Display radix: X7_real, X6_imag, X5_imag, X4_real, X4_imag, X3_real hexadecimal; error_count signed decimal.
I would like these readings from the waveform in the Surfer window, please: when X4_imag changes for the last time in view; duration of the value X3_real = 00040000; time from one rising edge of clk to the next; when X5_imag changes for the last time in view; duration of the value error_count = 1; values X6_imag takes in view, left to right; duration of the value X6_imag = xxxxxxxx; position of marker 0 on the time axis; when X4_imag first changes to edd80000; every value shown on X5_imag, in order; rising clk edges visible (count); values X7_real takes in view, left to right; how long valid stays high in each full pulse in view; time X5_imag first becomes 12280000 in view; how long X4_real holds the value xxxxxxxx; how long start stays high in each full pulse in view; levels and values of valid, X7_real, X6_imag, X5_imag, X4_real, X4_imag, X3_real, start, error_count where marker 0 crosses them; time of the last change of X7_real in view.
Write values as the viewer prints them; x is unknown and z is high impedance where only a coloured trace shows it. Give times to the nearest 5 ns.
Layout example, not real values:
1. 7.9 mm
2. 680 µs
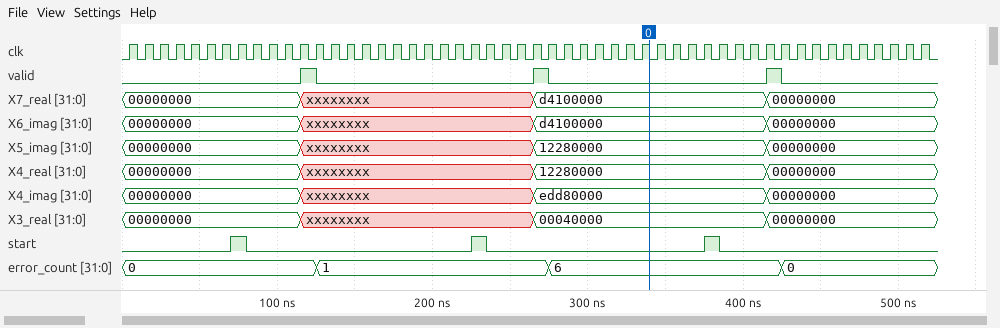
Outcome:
1. 415 ns
2. 150 ns
3. 10 ns
4. 415 ns
5. 150 ns
6. 00000000, xxxxxxxx, d4100000, 00000000
7. 150 ns
8. 340 ns
9. 265 ns
10. 00000000, xxxxxxxx, 12280000, 00000000
11. 52
12. 00000000, xxxxxxxx, d4100000, 00000000
13. 10 ns, 10 ns, 10 ns
14. 265 ns
15. 150 ns
16. 10 ns, 10 ns, 10 ns
17. valid=0, X7_real=d4100000, X6_imag=d4100000, X5_imag=12280000, X4_real=12280000, X4_imag=edd80000, X3_real=00040000, start=0, error_count=6
18. 415 ns
